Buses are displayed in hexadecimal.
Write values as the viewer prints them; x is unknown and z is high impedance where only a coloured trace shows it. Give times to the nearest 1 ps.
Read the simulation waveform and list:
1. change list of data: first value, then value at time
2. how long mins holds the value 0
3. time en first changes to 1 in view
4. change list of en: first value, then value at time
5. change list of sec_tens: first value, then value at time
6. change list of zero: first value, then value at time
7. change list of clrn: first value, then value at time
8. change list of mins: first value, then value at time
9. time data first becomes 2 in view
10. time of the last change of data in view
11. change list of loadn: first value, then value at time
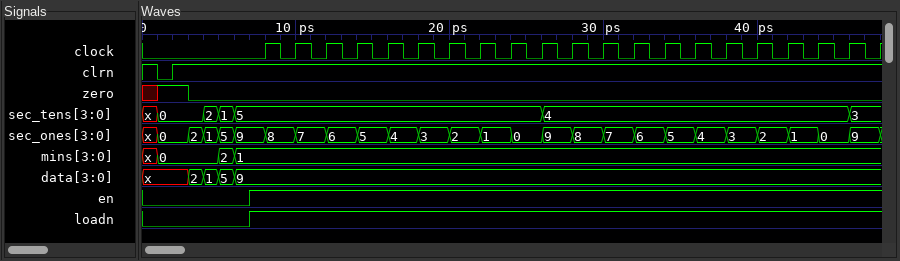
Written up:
x, 2 at 3 ps, 1 at 4 ps, 5 at 5 ps, 9 at 6 ps
4 ps
7 ps
0, 1 at 7 ps
x, 0 at 1 ps, 2 at 4 ps, 1 at 5 ps, 5 at 6 ps, 4 at 26 ps, 3 at 46 ps
x, 1 at 1 ps, 0 at 3 ps
1, 0 at 1 ps, 1 at 2 ps
x, 0 at 1 ps, 2 at 5 ps, 1 at 6 ps
3 ps
6 ps
0, 1 at 7 ps
